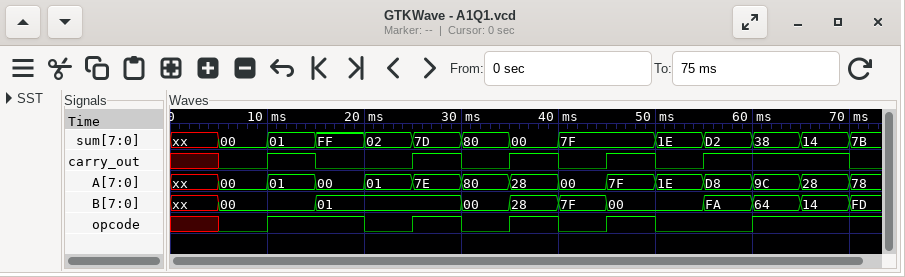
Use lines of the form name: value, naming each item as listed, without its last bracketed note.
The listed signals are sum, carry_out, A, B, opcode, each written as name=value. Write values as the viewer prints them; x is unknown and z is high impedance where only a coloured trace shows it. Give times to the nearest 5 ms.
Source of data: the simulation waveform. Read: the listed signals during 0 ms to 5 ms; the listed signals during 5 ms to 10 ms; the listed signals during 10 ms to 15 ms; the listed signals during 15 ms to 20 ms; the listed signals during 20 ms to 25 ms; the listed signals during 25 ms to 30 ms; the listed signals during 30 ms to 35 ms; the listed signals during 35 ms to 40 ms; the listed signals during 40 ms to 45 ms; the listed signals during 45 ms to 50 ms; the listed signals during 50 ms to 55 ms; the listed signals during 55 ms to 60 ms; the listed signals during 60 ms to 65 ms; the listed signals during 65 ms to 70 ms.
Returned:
the listed signals during 0 ms to 5 ms: sum=xx, carry_out=x, A=xx, B=xx, opcode=x
the listed signals during 5 ms to 10 ms: sum=00, carry_out=0, A=00, B=00, opcode=0
the listed signals during 10 ms to 15 ms: sum=01, carry_out=1, A=01, B=00, opcode=1
the listed signals during 15 ms to 20 ms: sum=FF, carry_out=0, A=00, B=01, opcode=1
the listed signals during 20 ms to 25 ms: sum=02, carry_out=0, A=01, B=01, opcode=0
the listed signals during 25 ms to 30 ms: sum=7D, carry_out=1, A=7E, B=01, opcode=1
the listed signals during 30 ms to 35 ms: sum=80, carry_out=0, A=80, B=00, opcode=0
the listed signals during 35 ms to 40 ms: sum=00, carry_out=1, A=28, B=28, opcode=1
the listed signals during 40 ms to 45 ms: sum=7F, carry_out=0, A=00, B=7F, opcode=0
the listed signals during 45 ms to 50 ms: sum=7F, carry_out=1, A=7F, B=00, opcode=1
the listed signals during 50 ms to 55 ms: sum=1E, carry_out=0, A=1E, B=00, opcode=0
the listed signals during 55 ms to 60 ms: sum=D2, carry_out=1, A=D8, B=FA, opcode=0
the listed signals during 60 ms to 65 ms: sum=38, carry_out=1, A=9C, B=64, opcode=1
the listed signals during 65 ms to 70 ms: sum=14, carry_out=1, A=28, B=14, opcode=1
